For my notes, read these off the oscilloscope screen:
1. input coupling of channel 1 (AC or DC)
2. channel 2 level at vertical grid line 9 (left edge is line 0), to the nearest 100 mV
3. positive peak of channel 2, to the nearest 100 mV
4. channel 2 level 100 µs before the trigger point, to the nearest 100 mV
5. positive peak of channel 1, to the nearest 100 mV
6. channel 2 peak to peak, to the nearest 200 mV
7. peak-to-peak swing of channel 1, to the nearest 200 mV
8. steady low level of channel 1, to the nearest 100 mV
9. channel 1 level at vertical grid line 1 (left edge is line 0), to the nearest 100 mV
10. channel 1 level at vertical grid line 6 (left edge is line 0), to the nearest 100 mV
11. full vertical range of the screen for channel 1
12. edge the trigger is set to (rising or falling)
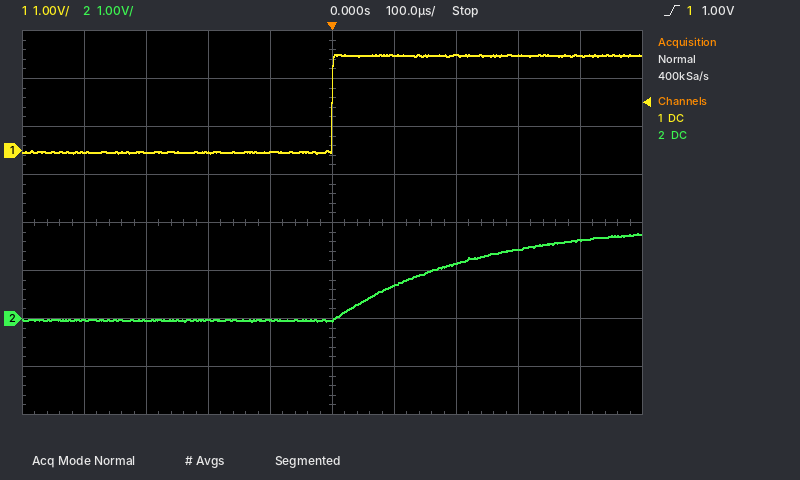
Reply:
DC
1.6 V
1.8 V
0.0 V
2.0 V
1.8 V
2.0 V
0.0 V
0.0 V
2.0 V
8 V
rising
